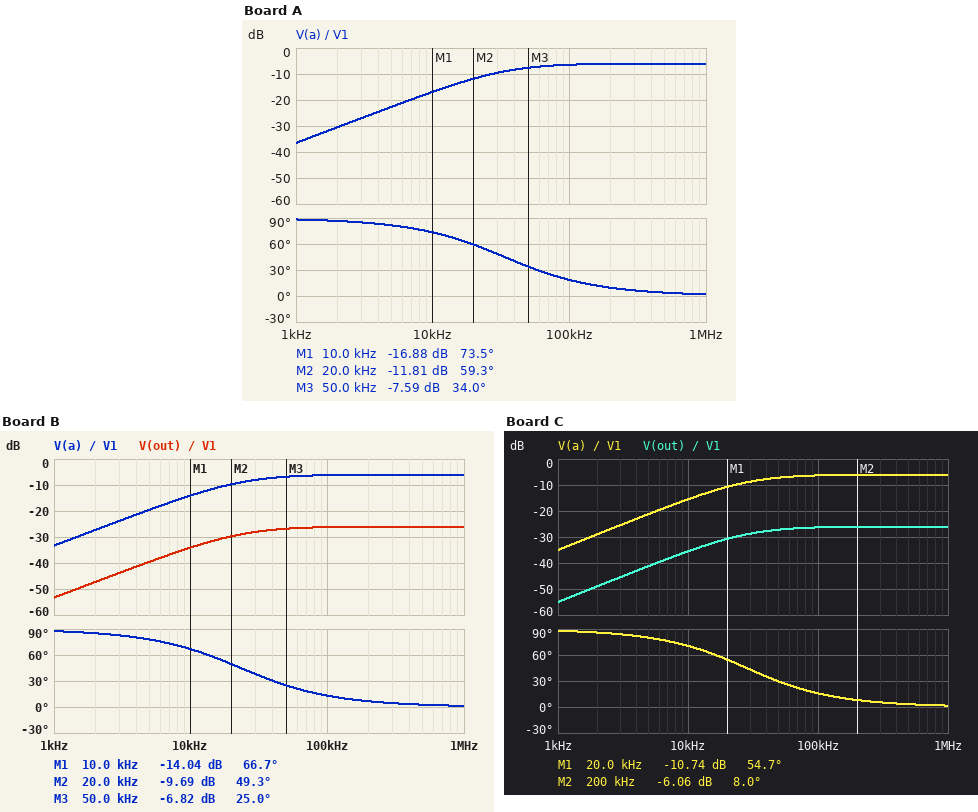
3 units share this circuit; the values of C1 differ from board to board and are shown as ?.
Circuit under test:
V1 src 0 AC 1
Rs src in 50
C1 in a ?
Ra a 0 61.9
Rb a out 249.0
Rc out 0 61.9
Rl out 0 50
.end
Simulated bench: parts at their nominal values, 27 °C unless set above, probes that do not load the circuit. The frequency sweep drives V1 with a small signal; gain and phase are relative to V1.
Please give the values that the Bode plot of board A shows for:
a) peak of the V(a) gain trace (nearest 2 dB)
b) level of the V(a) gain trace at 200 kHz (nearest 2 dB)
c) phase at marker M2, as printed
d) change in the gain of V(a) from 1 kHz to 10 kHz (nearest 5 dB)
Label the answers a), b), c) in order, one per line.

a) -6 dB
b) -6 dB
c) 59.3 deg
d) 20 dB
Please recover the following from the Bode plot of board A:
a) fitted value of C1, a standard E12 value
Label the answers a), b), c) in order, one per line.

a) 47 nF
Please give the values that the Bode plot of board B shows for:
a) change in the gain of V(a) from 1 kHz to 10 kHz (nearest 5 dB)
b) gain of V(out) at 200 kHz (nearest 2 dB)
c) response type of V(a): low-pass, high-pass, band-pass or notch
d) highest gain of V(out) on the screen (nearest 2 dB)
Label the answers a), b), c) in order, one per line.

a) 20 dB
b) -26 dB
c) high-pass
d) -26 dB
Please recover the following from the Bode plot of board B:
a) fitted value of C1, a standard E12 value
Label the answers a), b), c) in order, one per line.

a) 68 nF
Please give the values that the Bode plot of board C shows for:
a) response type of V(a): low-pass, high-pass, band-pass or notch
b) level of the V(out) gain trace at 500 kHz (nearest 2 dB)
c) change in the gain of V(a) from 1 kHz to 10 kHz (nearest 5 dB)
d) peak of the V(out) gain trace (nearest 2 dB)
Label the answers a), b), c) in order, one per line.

a) high-pass
b) -26 dB
c) 20 dB
d) -26 dB
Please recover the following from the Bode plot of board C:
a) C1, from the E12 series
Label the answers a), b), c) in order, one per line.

a) 56 nF
